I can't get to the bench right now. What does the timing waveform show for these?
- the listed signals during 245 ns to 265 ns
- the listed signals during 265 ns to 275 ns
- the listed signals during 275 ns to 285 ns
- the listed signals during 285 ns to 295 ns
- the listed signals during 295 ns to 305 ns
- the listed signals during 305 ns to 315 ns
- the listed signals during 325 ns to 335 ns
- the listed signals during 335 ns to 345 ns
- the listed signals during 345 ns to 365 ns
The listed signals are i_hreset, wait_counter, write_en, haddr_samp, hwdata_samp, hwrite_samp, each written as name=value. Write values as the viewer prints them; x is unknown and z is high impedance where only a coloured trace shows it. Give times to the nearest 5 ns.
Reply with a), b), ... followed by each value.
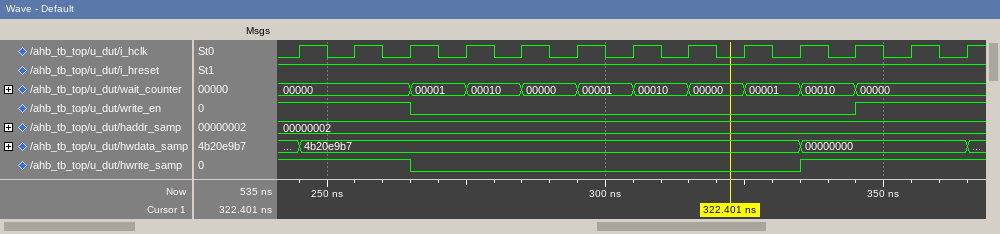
a) i_hreset=1, wait_counter=00000, write_en=1, haddr_samp=00000002, hwdata_samp=4b20e9b7, hwrite_samp=1
b) i_hreset=1, wait_counter=00001, write_en=0, haddr_samp=00000002, hwdata_samp=4b20e9b7, hwrite_samp=0
c) i_hreset=1, wait_counter=00010, write_en=0, haddr_samp=00000002, hwdata_samp=4b20e9b7, hwrite_samp=0
d) i_hreset=1, wait_counter=00000, write_en=0, haddr_samp=00000002, hwdata_samp=4b20e9b7, hwrite_samp=0
e) i_hreset=1, wait_counter=00001, write_en=0, haddr_samp=00000002, hwdata_samp=4b20e9b7, hwrite_samp=0
f) i_hreset=1, wait_counter=00010, write_en=0, haddr_samp=00000002, hwdata_samp=4b20e9b7, hwrite_samp=0
g) i_hreset=1, wait_counter=00001, write_en=0, haddr_samp=00000002, hwdata_samp=4b20e9b7, hwrite_samp=0
h) i_hreset=1, wait_counter=00010, write_en=0, haddr_samp=00000002, hwdata_samp=00000000, hwrite_samp=1
i) i_hreset=1, wait_counter=00000, write_en=1, haddr_samp=00000002, hwdata_samp=00000000, hwrite_samp=1
